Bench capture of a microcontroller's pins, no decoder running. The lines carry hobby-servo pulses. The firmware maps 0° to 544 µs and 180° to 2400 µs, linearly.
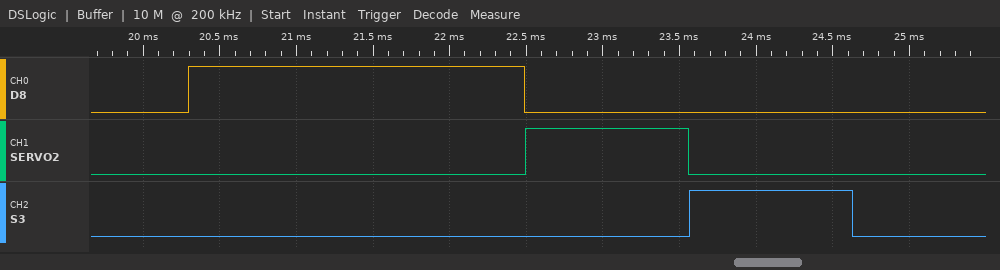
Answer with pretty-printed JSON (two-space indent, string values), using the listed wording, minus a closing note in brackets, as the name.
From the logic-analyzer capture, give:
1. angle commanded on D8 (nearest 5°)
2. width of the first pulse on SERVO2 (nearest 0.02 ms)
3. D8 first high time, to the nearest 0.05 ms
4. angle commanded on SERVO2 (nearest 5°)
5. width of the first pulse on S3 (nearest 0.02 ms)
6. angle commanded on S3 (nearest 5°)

{
  "angle commanded on D8": "160°",
  "width of the first pulse on SERVO2": "1.06 ms",
  "D8 first high time, to the nearest 0.05 ms": "2.20 ms",
  "angle commanded on SERVO2": "50°",
  "width of the first pulse on S3": "1.06 ms",
  "angle commanded on S3": "50°"
}
